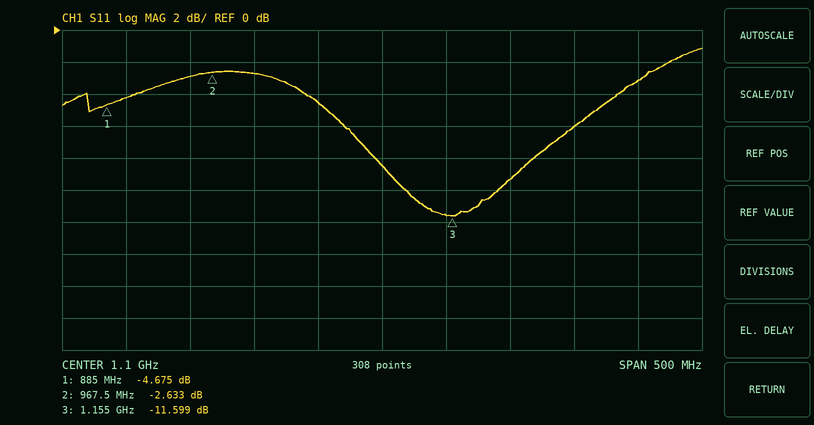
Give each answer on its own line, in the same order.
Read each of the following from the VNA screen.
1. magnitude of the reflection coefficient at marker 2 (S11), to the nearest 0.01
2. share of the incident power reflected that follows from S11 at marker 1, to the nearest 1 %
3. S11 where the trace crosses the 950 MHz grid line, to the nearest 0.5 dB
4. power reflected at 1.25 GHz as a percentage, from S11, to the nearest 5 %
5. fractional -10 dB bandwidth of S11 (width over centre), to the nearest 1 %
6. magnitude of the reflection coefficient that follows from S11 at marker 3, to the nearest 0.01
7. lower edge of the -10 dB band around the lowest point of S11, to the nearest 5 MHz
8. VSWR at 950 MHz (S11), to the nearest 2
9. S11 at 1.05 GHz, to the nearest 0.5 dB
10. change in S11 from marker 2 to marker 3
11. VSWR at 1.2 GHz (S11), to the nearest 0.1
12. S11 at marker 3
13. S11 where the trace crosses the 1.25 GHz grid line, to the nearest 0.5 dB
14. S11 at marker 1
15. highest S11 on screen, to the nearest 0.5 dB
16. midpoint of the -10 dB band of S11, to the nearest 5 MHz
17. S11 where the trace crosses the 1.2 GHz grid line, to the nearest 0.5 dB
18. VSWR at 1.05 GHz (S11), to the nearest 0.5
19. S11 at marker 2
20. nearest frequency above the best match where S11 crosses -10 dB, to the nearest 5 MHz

0.74
34 %
-3.0 dB
25 %
6 %
0.26
1.120 GHz
6
-4.5 dB
-8.966 dB
2.0
-11.599 dB
-6.0 dB
-4.675 dB
-1.0 dB
1.155 GHz
-9.5 dB
4.0
-2.633 dB
1.190 GHz
